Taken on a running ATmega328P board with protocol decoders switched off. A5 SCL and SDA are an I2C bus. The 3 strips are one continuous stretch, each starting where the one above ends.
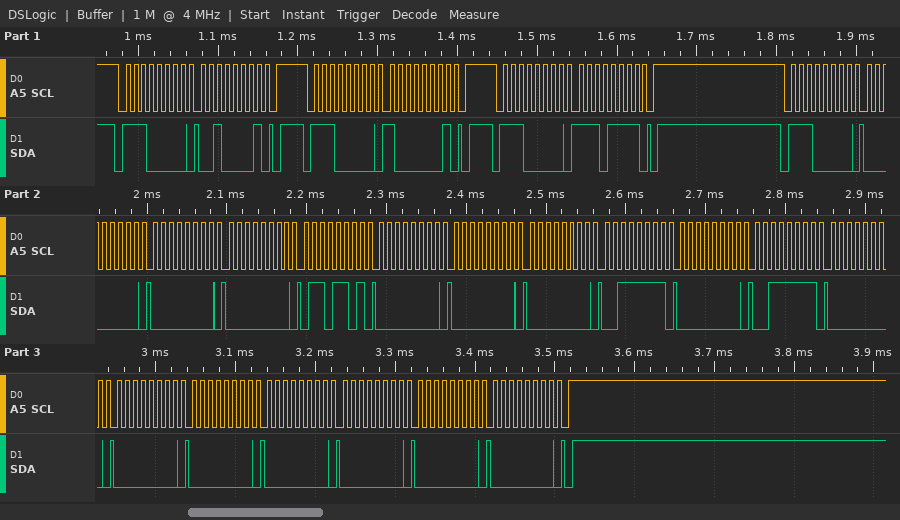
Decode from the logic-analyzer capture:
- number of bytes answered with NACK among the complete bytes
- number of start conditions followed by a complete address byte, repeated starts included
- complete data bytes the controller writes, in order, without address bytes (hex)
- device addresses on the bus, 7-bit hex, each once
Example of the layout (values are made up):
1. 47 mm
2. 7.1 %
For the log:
1. 0
2. 4
3. 21 81 EF 00 00 00 6D 00 00 00 3F 00 3F 00 00 00 00 00 00 00
4. 0x70
